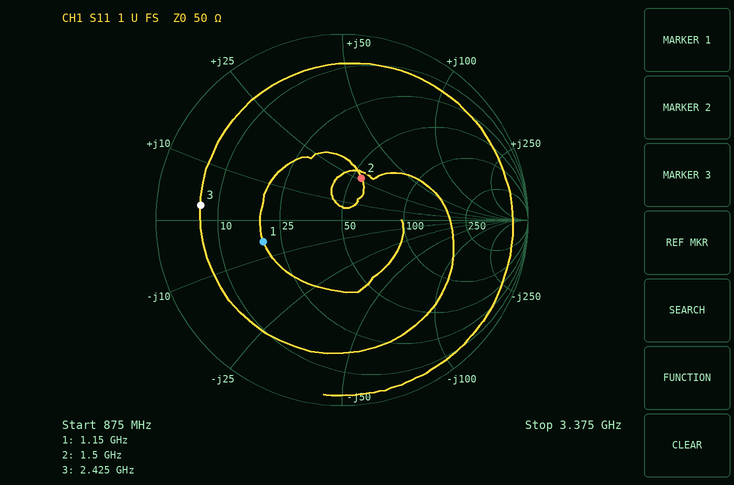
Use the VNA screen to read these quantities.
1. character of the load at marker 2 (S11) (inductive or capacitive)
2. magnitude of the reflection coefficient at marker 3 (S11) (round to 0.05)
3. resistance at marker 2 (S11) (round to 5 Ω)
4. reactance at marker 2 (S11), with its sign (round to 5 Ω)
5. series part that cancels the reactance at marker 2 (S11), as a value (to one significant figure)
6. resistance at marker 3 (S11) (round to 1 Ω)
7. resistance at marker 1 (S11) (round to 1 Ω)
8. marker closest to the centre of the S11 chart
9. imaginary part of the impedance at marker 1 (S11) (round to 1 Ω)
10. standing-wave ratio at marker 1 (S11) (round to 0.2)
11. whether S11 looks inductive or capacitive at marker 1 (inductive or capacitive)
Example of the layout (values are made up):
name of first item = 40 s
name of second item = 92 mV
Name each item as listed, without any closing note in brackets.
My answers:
character of the load at marker 2 (S11) = inductive
magnitude of the reflection coefficient at marker 3 (S11) = 0.75
resistance at marker 2 (S11) = 55 Ω
reactance at marker 2 (S11), with its sign = +25 Ω
series part that cancels the reactance at marker 2 (S11), as a value = 4 pF
resistance at marker 3 (S11) = 7 Ω
resistance at marker 1 (S11) = 20 Ω
marker closest to the centre of the S11 chart = marker 2
imaginary part of the impedance at marker 1 (S11) = -6 Ω
standing-wave ratio at marker 1 (S11) = 2.6
whether S11 looks inductive or capacitive at marker 1 = capacitive
